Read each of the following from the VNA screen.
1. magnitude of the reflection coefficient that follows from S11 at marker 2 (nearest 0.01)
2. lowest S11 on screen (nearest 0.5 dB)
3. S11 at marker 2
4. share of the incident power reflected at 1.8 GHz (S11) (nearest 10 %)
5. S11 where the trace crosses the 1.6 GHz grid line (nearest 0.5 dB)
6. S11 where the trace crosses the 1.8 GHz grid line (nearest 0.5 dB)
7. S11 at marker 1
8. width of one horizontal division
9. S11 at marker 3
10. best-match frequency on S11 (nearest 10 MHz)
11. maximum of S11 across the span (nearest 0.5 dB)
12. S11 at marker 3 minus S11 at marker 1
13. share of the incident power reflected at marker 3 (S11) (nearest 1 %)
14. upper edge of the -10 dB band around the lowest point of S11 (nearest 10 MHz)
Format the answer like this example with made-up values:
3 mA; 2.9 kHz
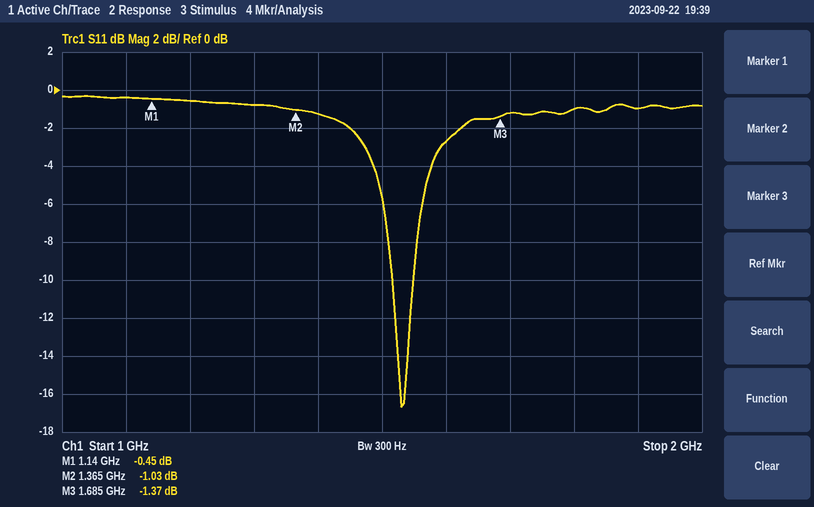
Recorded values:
0.89; -16.5 dB; -1.03 dB; 80 %; -2.5 dB; -1.0 dB; -0.45 dB; 100 MHz; -1.37 dB; 1.53 GHz; -0.5 dB; -0.92 dB; 73 %; 1.55 GHz
